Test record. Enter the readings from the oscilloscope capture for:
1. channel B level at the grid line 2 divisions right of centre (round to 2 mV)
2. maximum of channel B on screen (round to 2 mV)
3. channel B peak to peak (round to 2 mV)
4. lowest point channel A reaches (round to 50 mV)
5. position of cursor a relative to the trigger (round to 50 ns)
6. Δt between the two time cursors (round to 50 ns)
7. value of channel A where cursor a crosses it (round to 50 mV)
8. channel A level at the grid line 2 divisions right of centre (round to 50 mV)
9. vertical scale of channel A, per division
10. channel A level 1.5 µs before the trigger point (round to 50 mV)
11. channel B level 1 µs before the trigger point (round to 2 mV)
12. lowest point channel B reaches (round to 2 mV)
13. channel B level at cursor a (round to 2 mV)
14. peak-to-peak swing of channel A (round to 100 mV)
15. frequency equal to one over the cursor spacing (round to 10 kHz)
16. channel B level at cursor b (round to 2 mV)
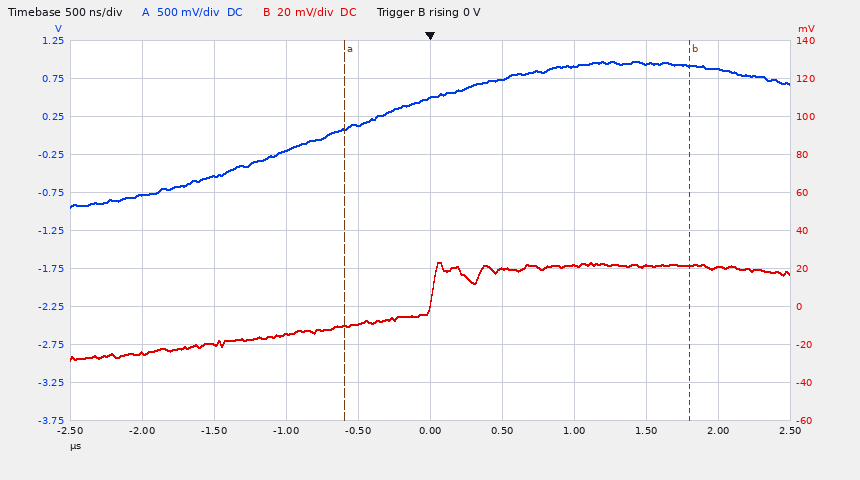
22 mV
24 mV
52 mV
-950 mV
-600 ns
2.40 µs
100 mV
900 mV
500 mV
-550 mV
-14 mV
-28 mV
-10 mV
1.90 V
420 kHz
22 mV
